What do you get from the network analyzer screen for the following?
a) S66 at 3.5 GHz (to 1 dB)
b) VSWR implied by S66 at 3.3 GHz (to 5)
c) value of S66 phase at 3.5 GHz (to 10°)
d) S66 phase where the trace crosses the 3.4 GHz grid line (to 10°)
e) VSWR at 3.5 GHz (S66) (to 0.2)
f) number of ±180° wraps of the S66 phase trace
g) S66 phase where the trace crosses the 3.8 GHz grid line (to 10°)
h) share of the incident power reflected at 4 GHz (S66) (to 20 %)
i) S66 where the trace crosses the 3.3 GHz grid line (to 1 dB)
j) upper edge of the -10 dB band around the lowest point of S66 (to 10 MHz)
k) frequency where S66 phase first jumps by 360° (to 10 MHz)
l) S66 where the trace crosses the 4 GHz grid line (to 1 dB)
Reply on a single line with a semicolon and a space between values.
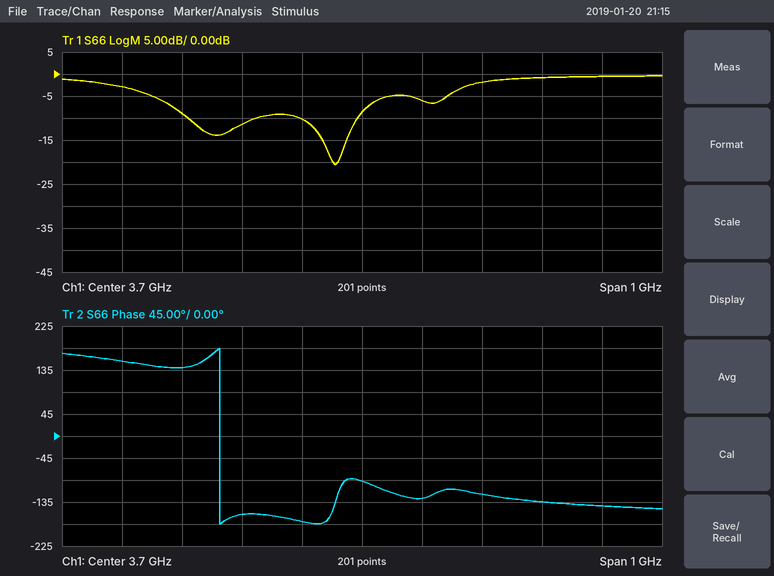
-11 dB; 5; -160°; 140°; 1.8; 1; -130°; 80 %; -3 dB; 3.69 GHz; 3.46 GHz; -1 dB
